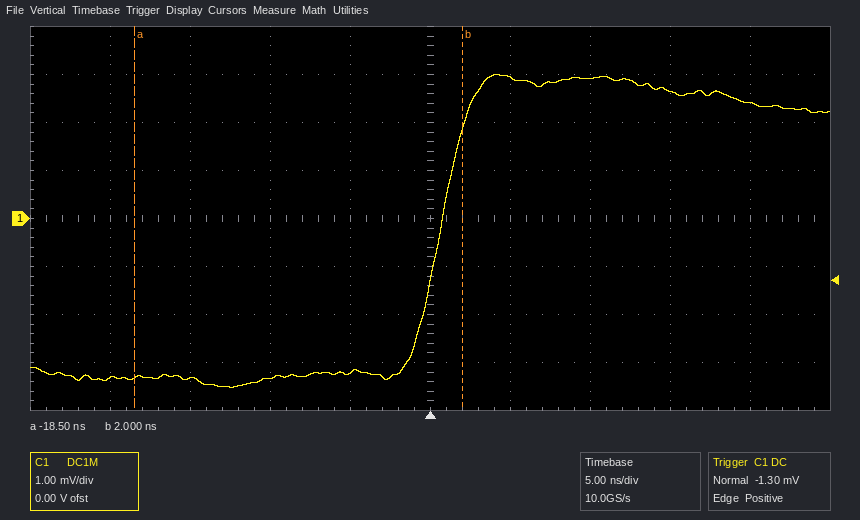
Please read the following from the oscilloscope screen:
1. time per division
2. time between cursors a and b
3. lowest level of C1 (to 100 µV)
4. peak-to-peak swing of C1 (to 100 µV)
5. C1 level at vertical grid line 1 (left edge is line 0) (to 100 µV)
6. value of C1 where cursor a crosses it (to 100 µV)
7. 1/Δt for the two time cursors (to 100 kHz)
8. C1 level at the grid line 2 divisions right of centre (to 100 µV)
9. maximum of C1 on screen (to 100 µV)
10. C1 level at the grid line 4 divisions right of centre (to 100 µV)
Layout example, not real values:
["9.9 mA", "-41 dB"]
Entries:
["5 ns", "20.5 ns", "-3.5 mV", "6.5 mV", "-3.3 mV", "-3.3 mV", "48.8 MHz", "2.9 mV", "3.0 mV", "2.4 mV"]
